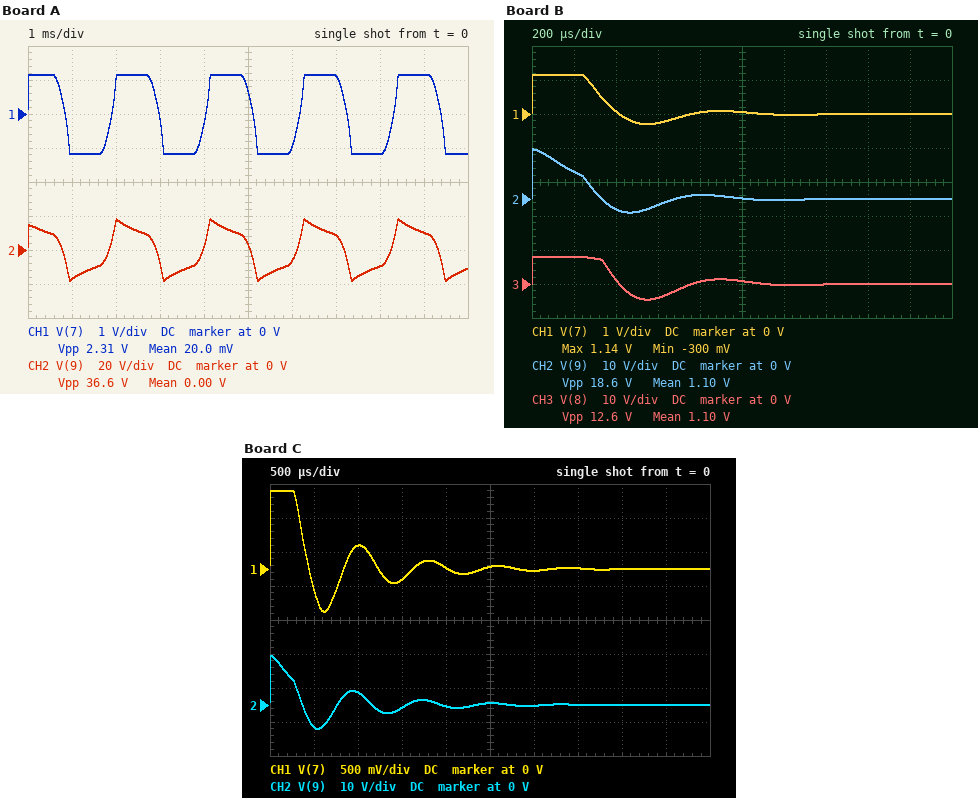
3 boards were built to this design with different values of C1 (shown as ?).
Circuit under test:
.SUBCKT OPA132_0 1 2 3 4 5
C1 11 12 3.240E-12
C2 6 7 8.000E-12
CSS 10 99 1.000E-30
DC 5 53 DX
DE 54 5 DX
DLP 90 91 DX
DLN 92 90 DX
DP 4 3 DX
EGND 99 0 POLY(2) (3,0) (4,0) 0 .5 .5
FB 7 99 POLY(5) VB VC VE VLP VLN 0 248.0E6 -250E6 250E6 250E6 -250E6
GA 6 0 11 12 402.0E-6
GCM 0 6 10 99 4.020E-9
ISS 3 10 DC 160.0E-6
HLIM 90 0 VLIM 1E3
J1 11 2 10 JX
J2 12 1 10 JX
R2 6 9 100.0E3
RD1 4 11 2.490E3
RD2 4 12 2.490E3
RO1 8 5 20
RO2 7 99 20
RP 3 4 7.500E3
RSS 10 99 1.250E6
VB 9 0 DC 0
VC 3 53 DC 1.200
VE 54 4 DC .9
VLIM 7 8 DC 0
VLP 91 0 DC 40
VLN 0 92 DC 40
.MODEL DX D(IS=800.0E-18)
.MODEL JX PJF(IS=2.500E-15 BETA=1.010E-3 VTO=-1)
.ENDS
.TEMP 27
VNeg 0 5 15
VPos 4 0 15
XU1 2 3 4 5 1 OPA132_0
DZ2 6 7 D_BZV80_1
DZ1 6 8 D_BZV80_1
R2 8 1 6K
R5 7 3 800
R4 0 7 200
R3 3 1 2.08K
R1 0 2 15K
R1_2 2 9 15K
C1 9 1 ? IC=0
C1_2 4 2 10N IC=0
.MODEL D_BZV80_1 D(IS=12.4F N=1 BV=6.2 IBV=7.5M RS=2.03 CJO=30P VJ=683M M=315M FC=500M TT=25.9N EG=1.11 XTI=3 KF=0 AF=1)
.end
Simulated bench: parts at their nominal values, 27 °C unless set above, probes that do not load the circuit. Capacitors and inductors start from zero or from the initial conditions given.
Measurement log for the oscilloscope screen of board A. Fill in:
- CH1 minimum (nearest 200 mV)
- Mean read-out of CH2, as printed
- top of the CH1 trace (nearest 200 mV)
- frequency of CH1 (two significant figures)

-1.2 V
0.00 V
1.2 V
470 Hz
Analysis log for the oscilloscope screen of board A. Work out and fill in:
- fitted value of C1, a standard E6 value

33 nF
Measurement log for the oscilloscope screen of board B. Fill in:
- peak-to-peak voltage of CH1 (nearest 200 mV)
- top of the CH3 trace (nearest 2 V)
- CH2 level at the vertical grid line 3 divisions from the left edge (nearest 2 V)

1.4 V
8 V
-2 V
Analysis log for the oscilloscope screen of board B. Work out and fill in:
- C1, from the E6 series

4.7 nF
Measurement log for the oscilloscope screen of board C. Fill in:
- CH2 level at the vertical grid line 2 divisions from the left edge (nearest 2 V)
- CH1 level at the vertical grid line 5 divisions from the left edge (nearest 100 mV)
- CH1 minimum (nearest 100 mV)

4 V
0 V
-600 mV
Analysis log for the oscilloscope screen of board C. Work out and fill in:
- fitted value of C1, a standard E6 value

6.8 nF
